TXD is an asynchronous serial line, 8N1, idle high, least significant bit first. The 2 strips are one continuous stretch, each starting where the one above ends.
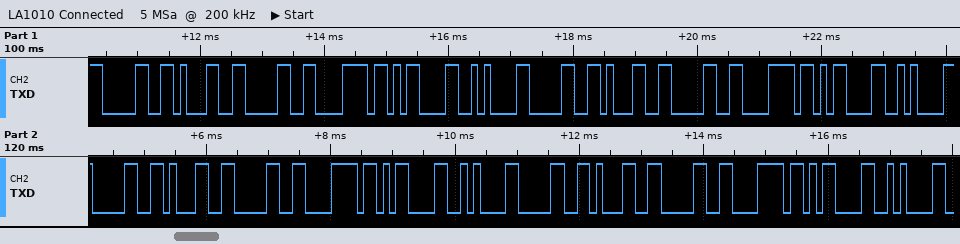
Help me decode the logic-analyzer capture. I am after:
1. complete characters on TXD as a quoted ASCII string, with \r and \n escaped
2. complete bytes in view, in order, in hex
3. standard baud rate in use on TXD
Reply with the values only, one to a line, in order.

"010x\r\n010x\r\n010x\r\n010x\r\n"
30 31 30 78 0D 0A 30 31 30 78 0D 0A 30 31 30 78 0D 0A 30 31 30 78 0D 0A
9600 baud
